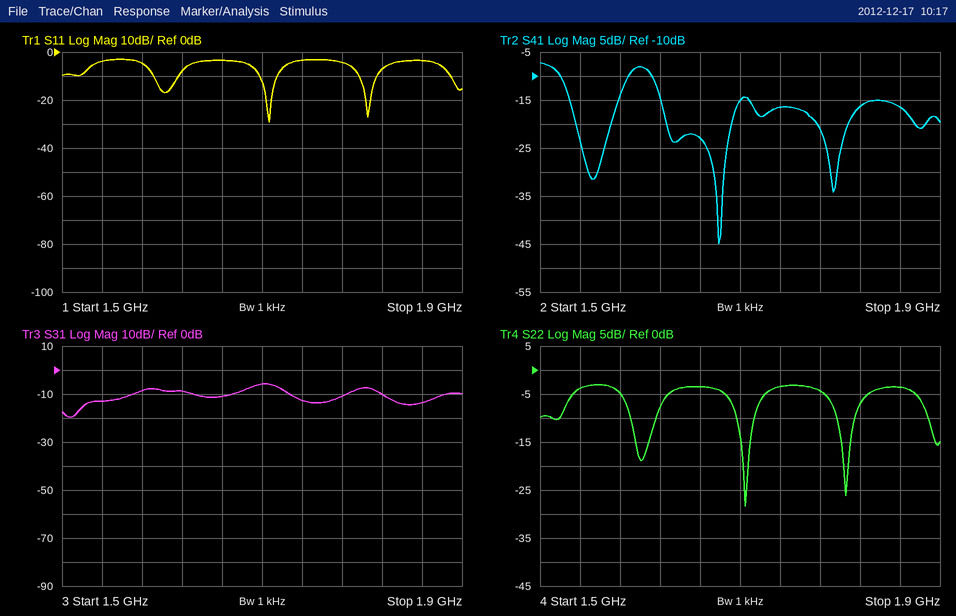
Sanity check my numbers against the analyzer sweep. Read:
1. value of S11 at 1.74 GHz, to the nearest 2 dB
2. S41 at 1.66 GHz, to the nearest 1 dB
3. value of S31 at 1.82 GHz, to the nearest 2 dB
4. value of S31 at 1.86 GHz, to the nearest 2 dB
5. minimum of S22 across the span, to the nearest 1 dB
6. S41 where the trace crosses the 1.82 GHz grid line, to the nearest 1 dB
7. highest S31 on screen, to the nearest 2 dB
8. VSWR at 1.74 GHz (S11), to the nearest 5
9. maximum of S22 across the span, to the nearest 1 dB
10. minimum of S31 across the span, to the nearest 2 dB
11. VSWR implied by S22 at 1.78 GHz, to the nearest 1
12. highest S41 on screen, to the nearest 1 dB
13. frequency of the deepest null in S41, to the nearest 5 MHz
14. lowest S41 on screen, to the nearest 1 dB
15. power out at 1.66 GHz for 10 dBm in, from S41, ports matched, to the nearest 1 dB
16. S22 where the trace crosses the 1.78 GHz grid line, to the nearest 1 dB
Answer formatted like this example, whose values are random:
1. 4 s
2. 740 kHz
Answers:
1. -4 dB
2. -23 dB
3. -10 dB
4. -14 dB
5. -28 dB
6. -16 dB
7. -6 dB
8. 5
9. -3 dB
10. -20 dB
11. 4
12. -7 dB
13. 1.680 GHz
14. -45 dB
15. -13 dBm
16. -4 dB
